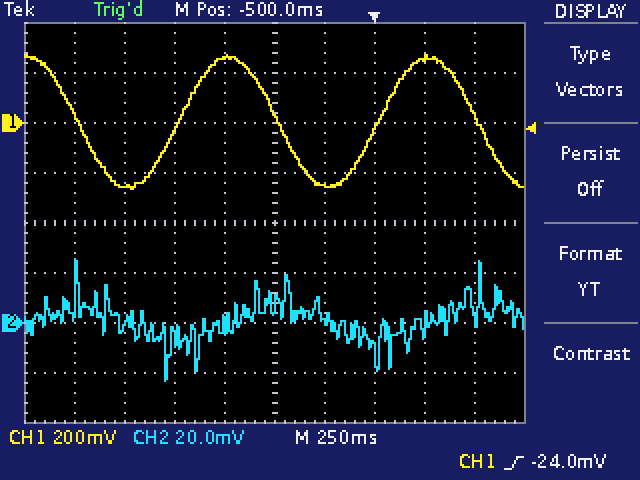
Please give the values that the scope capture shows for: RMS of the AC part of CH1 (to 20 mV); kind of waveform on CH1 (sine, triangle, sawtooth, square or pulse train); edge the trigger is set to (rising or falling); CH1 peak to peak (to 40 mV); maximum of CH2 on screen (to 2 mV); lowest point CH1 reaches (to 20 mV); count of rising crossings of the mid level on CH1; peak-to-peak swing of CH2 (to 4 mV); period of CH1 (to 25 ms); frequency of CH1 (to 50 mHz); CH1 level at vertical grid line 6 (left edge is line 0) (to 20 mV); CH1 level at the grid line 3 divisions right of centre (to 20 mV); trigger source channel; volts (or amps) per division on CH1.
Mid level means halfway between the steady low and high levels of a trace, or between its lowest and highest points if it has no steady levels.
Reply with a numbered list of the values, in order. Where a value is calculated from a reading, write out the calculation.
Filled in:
1. 520 mV / (2√2) ≈ 184 mV, so 180 mV to the nearest 20 mV
2. sine
3. rising
4. 520 mV
5. 26 mV
6. -260 mV
7. 2
8. 48 mV
9. 1.000 s
10. 1 / 1.000 s ≈ 1.00 Hz
11. -260 mV
12. 260 mV
13. CH1
14. 200 mV
